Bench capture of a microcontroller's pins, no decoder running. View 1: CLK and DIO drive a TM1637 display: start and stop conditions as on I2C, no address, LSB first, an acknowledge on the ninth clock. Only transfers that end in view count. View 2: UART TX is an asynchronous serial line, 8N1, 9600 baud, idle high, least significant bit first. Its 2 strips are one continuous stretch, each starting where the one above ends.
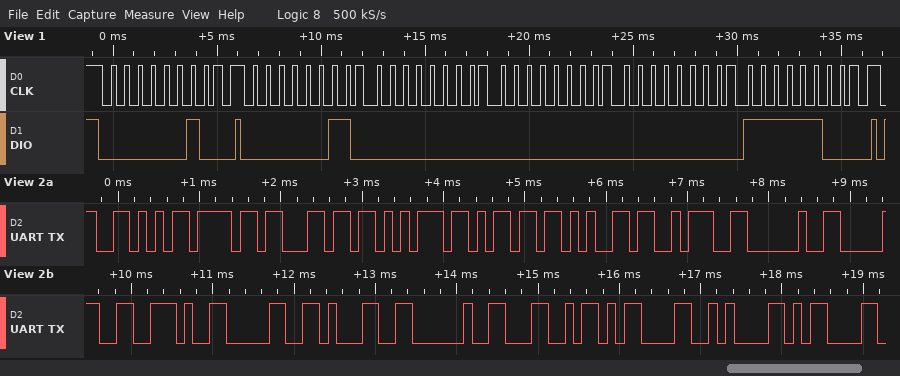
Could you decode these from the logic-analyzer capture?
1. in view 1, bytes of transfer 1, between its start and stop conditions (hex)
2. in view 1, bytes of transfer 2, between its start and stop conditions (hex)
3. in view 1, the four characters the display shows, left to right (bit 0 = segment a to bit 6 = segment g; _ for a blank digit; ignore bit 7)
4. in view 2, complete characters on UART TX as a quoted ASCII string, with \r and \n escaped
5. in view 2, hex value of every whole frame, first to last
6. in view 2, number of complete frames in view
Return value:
40
C0 00 00 00 3F
___0
"Volume: 0.01 L\r\n\r"
56 6F 6C 75 6D 65 3A 20 30 2E 30 31 20 4C 0D 0A 0D
17
